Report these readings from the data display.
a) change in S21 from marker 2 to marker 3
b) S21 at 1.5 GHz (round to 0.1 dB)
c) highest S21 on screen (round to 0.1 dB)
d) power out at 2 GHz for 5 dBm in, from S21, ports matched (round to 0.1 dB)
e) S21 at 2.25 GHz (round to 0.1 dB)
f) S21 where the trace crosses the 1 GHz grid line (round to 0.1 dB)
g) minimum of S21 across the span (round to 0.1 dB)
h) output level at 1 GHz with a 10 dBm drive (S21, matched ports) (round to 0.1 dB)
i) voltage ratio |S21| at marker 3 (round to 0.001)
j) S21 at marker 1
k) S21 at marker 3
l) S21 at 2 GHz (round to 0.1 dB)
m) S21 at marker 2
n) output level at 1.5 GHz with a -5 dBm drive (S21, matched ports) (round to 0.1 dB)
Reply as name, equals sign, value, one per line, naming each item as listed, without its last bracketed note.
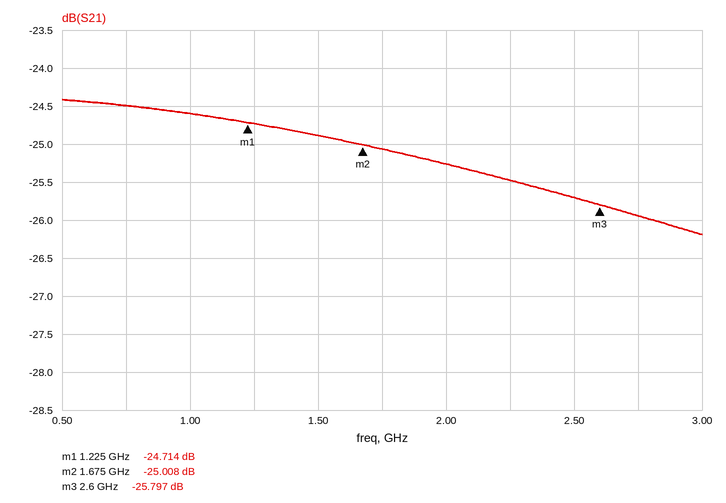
change in S21 from marker 2 to marker 3 = -0.789 dB
S21 at 1.5 GHz = -24.9 dB
highest S21 on screen = -24.4 dB
power out at 2 GHz for 5 dBm in, from S21, ports matched = -20.3 dBm
S21 at 2.25 GHz = -25.5 dB
S21 where the trace crosses the 1 GHz grid line = -24.6 dB
minimum of S21 across the span = -26.2 dB
output level at 1 GHz with a 10 dBm drive (S21, matched ports) = -14.6 dBm
voltage ratio |S21| at marker 3 = 0.051
S21 at marker 1 = -24.714 dB
S21 at marker 3 = -25.797 dB
S21 at 2 GHz = -25.3 dB
S21 at marker 2 = -25.008 dB
output level at 1.5 GHz with a -5 dBm drive (S21, matched ports) = -29.9 dBm
